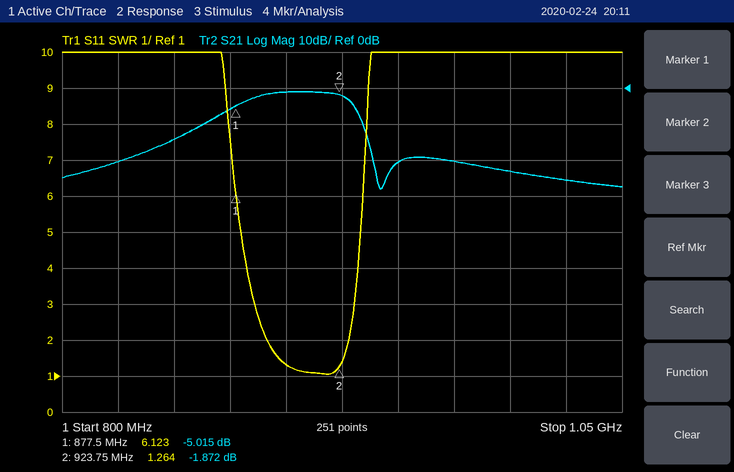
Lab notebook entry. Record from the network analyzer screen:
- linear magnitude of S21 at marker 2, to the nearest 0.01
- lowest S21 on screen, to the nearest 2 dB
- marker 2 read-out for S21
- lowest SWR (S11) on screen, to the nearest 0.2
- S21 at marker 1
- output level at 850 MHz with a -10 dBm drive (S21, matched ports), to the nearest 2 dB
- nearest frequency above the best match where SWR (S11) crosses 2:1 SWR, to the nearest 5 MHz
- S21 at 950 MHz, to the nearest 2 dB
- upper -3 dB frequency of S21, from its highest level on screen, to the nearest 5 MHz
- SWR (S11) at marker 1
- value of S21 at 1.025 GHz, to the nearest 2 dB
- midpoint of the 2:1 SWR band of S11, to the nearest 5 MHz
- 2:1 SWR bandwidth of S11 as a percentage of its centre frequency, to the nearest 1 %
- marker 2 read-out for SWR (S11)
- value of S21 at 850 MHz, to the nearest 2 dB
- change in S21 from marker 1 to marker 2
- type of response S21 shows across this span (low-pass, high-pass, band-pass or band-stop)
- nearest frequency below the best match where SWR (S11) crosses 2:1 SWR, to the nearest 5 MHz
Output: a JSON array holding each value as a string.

["0.81", "-28 dB", "-1.872 dB", "1.0", "-5.015 dB", "-24 dBm", "930 MHz", "-20 dB", "930 MHz", "6.123", "-26 dB", "910 MHz", "4 %", "1.264", "-14 dB", "3.143 dB", "band-pass", "890 MHz"]
